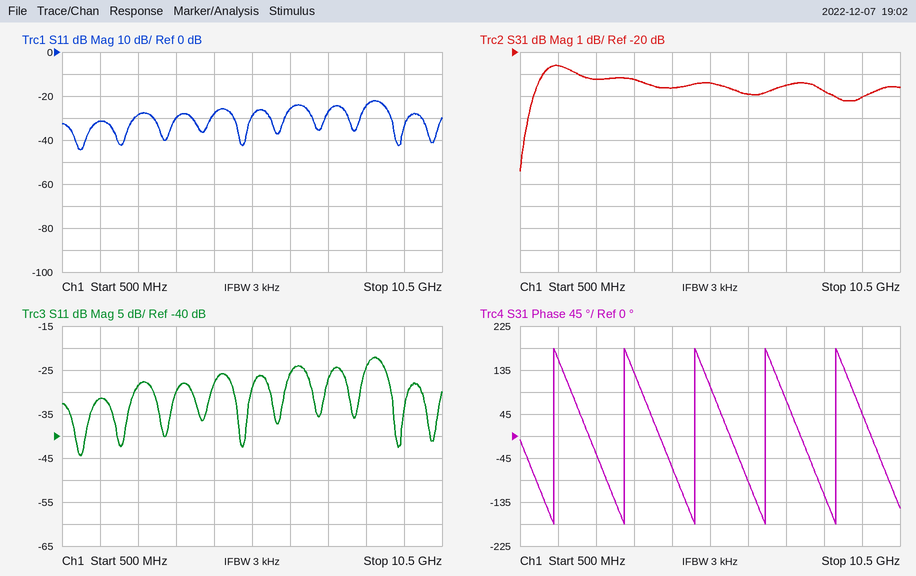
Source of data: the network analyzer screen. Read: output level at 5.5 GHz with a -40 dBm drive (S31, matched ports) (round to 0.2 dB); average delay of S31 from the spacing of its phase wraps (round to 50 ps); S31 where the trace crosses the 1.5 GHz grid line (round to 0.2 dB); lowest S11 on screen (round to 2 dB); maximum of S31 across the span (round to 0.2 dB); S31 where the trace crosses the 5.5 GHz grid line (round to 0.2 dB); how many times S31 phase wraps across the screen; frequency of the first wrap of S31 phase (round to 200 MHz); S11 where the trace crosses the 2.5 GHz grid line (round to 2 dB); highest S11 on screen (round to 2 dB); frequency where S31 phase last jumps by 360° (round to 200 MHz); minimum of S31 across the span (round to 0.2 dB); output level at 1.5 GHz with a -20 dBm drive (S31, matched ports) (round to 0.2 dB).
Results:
-61.4 dBm
550 ps
-20.6 dB
-44 dB
-20.6 dB
-21.4 dB
5
1.4 GHz
-28 dB
-22 dB
8.8 GHz
-25.4 dB
-40.6 dBm
